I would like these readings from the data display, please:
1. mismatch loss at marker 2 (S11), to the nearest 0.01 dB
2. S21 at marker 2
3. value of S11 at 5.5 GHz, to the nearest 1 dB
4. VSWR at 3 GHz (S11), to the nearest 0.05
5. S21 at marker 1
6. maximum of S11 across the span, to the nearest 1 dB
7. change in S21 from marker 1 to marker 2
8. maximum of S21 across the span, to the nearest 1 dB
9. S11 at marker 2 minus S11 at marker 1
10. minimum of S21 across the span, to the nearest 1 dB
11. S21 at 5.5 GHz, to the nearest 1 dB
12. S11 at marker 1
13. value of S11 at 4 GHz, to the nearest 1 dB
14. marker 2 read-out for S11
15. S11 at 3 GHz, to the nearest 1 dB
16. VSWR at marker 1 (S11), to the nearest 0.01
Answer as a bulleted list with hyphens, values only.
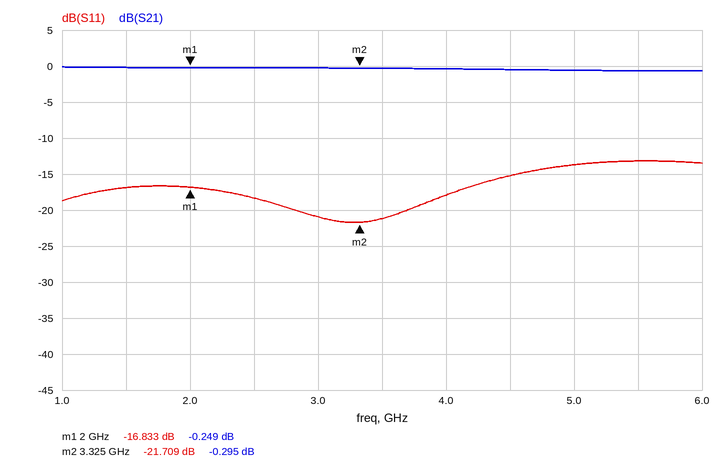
- 0.03 dB
- -0.295 dB
- -13 dB
- 1.20
- -0.249 dB
- -13 dB
- -0.046 dB
- 0 dB
- -4.876 dB
- -1 dB
- -1 dB
- -16.833 dB
- -18 dB
- -21.709 dB
- -21 dB
- 1.34
